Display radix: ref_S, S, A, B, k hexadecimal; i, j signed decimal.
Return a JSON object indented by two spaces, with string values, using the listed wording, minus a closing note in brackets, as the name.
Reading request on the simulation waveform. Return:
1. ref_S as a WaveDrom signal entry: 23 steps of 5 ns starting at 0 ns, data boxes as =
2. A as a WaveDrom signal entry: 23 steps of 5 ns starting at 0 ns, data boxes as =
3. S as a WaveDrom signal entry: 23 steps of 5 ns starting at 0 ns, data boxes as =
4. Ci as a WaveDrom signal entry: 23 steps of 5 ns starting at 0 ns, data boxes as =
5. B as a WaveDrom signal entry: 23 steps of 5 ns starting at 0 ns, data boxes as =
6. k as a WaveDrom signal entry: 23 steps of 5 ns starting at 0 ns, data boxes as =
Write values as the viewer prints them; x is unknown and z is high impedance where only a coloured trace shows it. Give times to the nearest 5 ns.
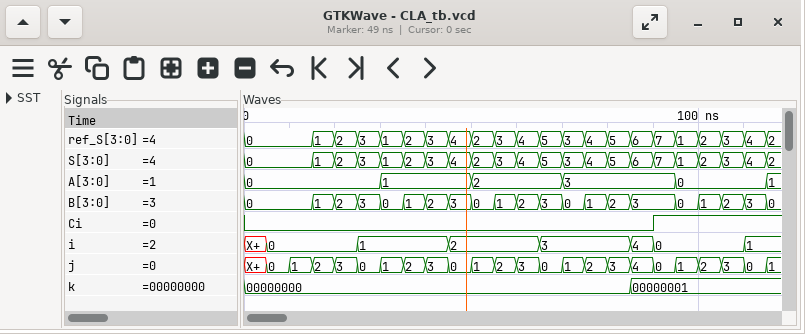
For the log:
{
  "ref_S as a WaveDrom signal entry: 23 steps of 5 ns starting at 0 ns, data boxes as =": "{name: 'ref_S', wave: '=..====================', data: '0 1 2 3 1 2 3 4 2 3 4 5 3 4 5 6 7 1 2 3 4'}",
  "A as a WaveDrom signal entry: 23 steps of 5 ns starting at 0 ns, data boxes as =": "{name: 'A', wave: '=.....=...=...=....=...', data: '0 1 2 3 0'}",
  "S as a WaveDrom signal entry: 23 steps of 5 ns starting at 0 ns, data boxes as =": "{name: 'S', wave: '=..====================', data: '0 1 2 3 1 2 3 4 2 3 4 5 3 4 5 6 7 1 2 3 4'}",
  "Ci as a WaveDrom signal entry: 23 steps of 5 ns starting at 0 ns, data boxes as =": "{name: 'Ci', wave: '0.................1....'}",
  "B as a WaveDrom signal entry: 23 steps of 5 ns starting at 0 ns, data boxes as =": "{name: 'B', wave: '=..===============.====', data: '0 1 2 3 0 1 2 3 0 1 2 3 0 1 2 3 0 1 2 3'}",
  "k as a WaveDrom signal entry: 23 steps of 5 ns starting at 0 ns, data boxes as =": "{name: 'k', wave: '=................=.....', data: '00000000 00000001'}"
}
